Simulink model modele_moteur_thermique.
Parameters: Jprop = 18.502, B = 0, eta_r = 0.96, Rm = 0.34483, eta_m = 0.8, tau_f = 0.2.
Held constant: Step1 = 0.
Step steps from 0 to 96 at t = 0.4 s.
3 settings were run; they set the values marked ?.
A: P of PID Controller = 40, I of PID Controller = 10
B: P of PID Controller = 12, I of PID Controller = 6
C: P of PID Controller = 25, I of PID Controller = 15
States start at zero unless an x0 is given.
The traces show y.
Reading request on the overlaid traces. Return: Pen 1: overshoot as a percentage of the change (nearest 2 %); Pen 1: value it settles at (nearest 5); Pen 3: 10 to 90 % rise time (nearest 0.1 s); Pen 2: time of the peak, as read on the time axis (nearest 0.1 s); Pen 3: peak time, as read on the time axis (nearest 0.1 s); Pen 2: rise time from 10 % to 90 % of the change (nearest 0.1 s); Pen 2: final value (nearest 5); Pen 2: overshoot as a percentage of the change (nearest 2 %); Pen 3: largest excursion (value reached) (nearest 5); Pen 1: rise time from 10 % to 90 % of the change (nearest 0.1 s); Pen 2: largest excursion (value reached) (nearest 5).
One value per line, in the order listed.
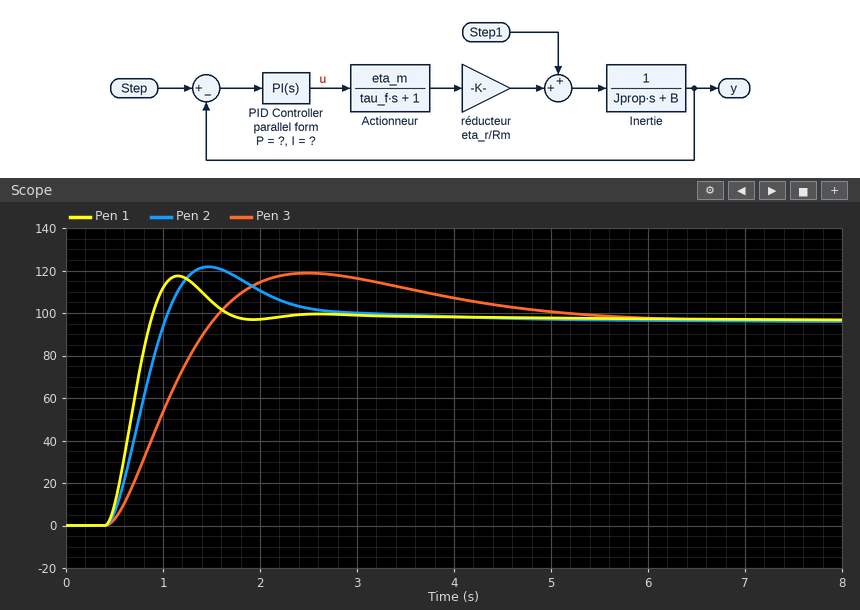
22 %
95
0.8 s
1.5 s
2.5 s
0.4 s
95
26 %
120
0.3 s
120
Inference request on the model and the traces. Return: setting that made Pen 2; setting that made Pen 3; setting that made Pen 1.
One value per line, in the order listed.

C
B
A
